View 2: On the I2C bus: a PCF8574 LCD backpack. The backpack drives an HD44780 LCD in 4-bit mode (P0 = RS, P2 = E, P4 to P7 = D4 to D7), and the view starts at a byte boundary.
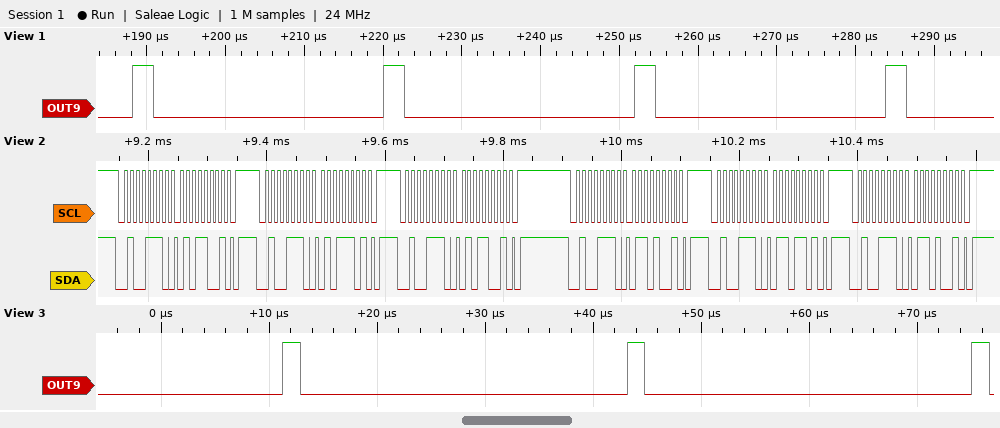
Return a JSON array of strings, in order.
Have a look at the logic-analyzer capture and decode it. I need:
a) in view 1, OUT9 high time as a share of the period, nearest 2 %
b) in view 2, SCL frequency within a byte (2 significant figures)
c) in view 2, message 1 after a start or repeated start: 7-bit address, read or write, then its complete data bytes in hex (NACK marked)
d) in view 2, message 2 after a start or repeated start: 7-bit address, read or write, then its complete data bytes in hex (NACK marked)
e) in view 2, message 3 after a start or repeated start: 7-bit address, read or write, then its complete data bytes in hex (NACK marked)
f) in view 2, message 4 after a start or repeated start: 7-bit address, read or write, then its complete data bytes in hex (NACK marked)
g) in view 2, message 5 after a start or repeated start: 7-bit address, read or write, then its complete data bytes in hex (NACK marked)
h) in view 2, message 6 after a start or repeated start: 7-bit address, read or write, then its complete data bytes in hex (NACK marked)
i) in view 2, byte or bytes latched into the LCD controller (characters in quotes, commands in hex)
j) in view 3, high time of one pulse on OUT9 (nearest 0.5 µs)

["8 %", "100 kHz", "0x27 write: 59", "0x27 write: 5D", "0x27 write: 59", "0x27 write: 69", "0x27 write: 6D", "0x27 write: 69", "'V'", "1.5 µs"]
